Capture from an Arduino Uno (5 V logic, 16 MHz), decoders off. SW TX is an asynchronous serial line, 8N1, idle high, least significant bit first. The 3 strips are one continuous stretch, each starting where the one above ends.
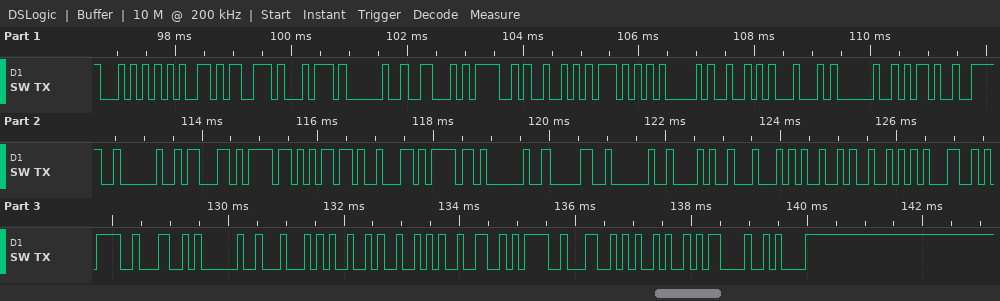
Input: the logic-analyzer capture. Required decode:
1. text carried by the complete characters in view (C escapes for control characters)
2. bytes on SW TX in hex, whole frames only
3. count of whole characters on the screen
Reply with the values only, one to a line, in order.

"Test FORWARD -> combo 0 (DIR1=L DIR2=L)\r\n"
0x54 0x65 0x73 0x74 0x20 0x46 0x4F 0x52 0x57 0x41 0x52 0x44 0x20 0x2D 0x3E 0x20 0x63 0x6F 0x6D 0x62 0x6F 0x20 0x30 0x20 0x28 0x44 0x49 0x52 0x31 0x3D 0x4C 0x20 0x44 0x49 0x52 0x32 0x3D 0x4C 0x29 0x0D 0x0A
41
